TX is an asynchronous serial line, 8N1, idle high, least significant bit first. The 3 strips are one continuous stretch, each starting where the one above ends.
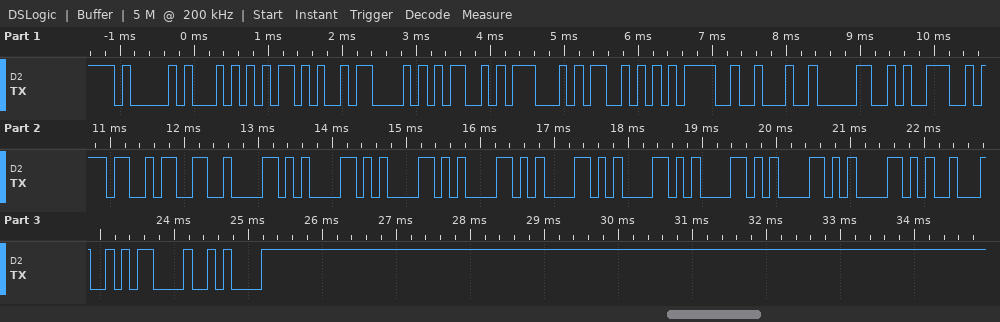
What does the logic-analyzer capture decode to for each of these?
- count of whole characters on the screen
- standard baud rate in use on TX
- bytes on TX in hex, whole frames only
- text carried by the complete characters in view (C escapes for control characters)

25
9600 baud
41 54 2B 43 4D 47 53 3D 22 30 39 37 33 58 58 58 58 58 58 58 58 58 22 0D 0A
"AT+CMGS=\"0973XXXXXXXXX\"\r\n"
